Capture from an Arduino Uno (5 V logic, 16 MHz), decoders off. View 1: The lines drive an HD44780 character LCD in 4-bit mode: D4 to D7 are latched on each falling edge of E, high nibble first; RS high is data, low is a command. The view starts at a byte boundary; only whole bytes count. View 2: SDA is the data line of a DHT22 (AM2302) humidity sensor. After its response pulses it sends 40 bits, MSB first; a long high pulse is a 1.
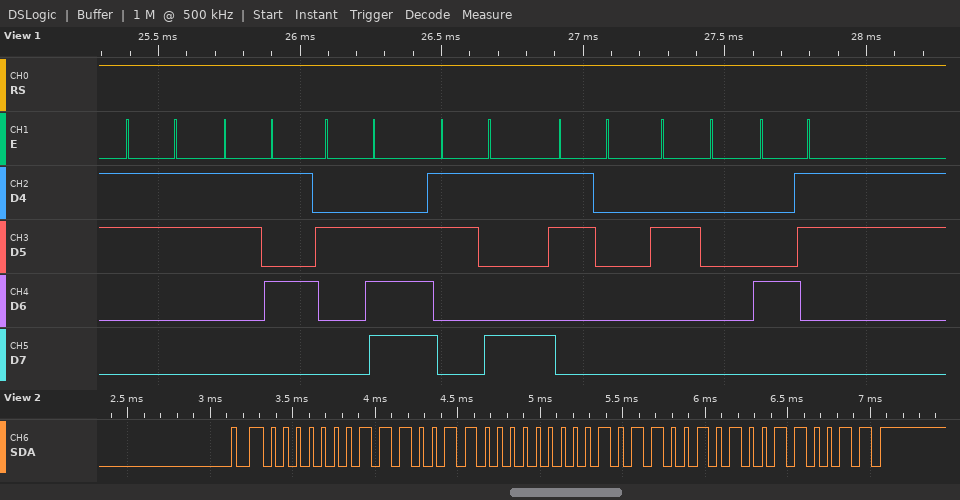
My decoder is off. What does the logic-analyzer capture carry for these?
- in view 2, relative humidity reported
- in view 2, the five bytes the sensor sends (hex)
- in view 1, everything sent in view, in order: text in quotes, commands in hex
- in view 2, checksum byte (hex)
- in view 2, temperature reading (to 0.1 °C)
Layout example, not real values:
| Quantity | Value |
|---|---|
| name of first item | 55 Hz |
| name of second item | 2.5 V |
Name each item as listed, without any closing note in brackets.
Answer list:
| Quantity | Value |
|---|---|
| in view 2, relative humidity reported | 46.0 % |
| in view 2, the five bytes the sensor sends | 01 CC 01 65 33 |
| in view 1, everything sent in view, in order: text in quotes, commands in hex | "35.90 C" |
| in view 2, checksum byte | 0x33 |
| in view 2, temperature reading | 35.7 °C |
